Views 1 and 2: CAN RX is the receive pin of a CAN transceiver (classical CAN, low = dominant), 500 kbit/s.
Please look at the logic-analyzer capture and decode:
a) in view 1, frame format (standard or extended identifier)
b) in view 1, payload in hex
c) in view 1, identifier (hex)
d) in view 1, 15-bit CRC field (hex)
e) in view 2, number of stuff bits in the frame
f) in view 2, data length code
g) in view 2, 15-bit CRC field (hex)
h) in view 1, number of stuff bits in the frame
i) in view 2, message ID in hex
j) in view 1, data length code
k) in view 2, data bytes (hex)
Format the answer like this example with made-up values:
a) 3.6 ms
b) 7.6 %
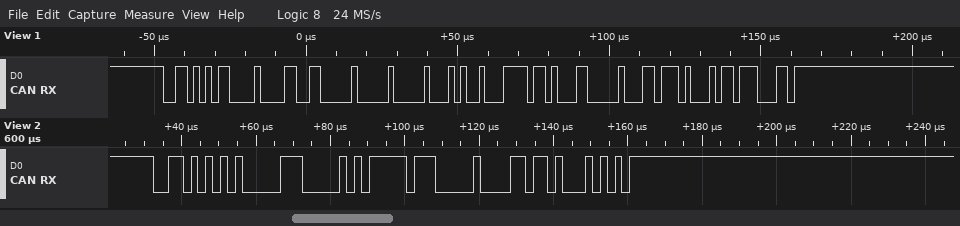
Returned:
a) standard
b) 66 00 00 52 3D A3 00 DD
c) 0x356
d) 0x0B71
e) 4
f) 3
g) 0x368A
h) 4
i) 0x355
j) 8
k) 02 FF 00
